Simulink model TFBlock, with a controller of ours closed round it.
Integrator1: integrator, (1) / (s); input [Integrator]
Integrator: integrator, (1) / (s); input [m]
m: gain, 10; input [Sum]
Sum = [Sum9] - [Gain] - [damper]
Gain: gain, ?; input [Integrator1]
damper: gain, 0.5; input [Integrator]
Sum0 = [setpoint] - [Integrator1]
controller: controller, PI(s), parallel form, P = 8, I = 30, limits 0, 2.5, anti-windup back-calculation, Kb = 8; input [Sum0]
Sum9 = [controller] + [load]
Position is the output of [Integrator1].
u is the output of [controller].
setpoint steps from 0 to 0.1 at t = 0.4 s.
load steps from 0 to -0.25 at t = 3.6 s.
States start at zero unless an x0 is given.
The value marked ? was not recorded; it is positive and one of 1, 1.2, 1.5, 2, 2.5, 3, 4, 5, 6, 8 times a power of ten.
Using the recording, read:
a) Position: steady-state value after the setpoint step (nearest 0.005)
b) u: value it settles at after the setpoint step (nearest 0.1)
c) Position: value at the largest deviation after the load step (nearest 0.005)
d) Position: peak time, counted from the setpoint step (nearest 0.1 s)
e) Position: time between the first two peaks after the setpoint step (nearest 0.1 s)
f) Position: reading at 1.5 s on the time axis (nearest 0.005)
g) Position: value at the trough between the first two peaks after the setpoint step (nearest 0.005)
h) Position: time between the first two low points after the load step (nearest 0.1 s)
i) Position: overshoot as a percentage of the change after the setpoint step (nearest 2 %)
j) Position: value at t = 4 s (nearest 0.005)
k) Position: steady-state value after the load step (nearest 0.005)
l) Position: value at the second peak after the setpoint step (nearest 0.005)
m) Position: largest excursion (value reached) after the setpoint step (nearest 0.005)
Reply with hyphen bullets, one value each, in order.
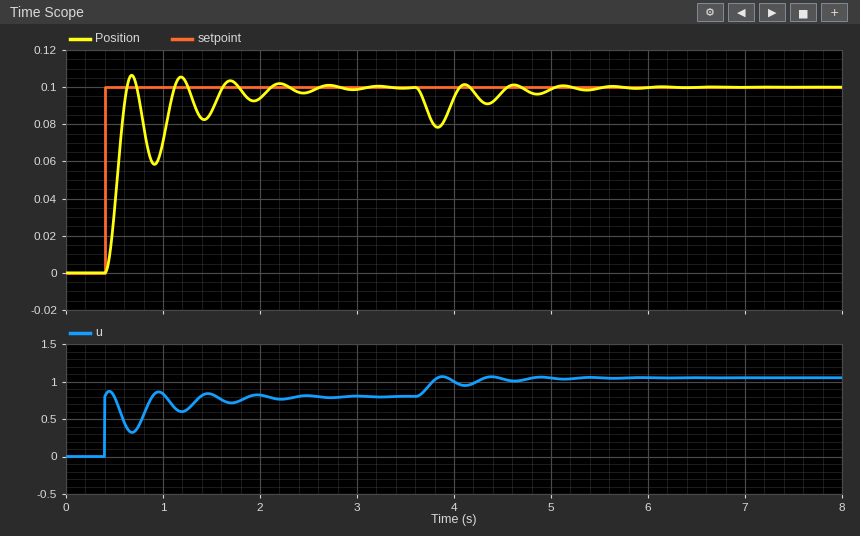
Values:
- 0.100
- 0.8
- 0.080
- 0.3 s
- 0.5 s
- 0.085
- 0.060
- 0.5 s
- 6 %
- 0.095
- 0.100
- 0.105
- 0.105
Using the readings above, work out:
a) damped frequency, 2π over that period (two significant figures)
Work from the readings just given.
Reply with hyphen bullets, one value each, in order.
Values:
- 13 rad/s
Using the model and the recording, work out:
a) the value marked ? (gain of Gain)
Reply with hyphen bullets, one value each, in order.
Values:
- 8
